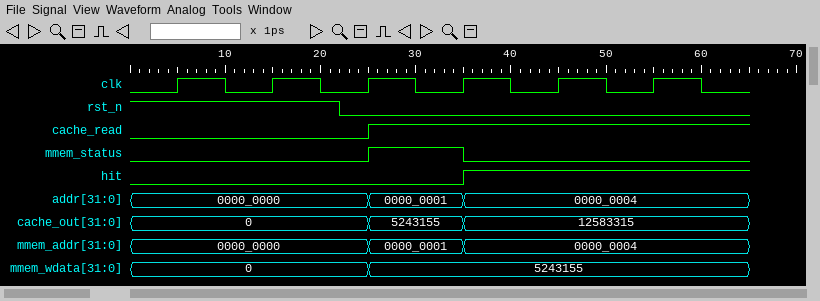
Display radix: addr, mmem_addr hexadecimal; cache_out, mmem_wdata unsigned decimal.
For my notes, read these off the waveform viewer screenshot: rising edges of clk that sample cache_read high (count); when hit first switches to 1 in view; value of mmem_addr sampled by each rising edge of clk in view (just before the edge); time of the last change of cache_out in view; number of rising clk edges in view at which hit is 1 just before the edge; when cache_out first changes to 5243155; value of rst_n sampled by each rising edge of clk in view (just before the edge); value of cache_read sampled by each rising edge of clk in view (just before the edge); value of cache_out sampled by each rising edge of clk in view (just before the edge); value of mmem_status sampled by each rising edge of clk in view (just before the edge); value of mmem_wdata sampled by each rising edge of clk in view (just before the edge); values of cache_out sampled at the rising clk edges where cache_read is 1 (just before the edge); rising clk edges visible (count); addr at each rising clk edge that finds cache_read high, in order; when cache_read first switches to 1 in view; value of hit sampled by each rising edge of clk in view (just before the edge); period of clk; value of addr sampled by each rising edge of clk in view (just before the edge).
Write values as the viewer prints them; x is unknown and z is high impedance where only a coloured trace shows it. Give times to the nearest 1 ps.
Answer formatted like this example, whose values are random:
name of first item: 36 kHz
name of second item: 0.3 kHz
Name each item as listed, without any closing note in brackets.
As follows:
rising edges of clk that sample cache_read high: 3
when hit first switches to 1 in view: 35 ps
value of mmem_addr sampled by each rising edge of clk in view: 0000_0000, 0000_0000, 0000_0000, 0000_0001, 0000_0004, 0000_0004
time of the last change of cache_out in view: 35 ps
number of rising clk edges in view at which hit is 1 just before the edge: 2
when cache_out first changes to 5243155: 25 ps
value of rst_n sampled by each rising edge of clk in view: 1 1 0 0 0 0
value of cache_read sampled by each rising edge of clk in view: 0 0 0 1 1 1
value of cache_out sampled by each rising edge of clk in view: 0, 0, 0, 5243155, 12583315, 12583315
value of mmem_status sampled by each rising edge of clk in view: 0 0 0 1 0 0
value of mmem_wdata sampled by each rising edge of clk in view: 0, 0, 0, 5243155, 5243155, 5243155
values of cache_out sampled at the rising clk edges where cache_read is 1: 5243155, 12583315, 12583315
rising clk edges visible: 6
addr at each rising clk edge that finds cache_read high, in order: 0000_0001, 0000_0004, 0000_0004
when cache_read first switches to 1 in view: 25 ps
value of hit sampled by each rising edge of clk in view: 0 0 0 0 1 1
period of clk: 10 ps
value of addr sampled by each rising edge of clk in view: 0000_0000, 0000_0000, 0000_0000, 0000_0001, 0000_0004, 0000_0004
